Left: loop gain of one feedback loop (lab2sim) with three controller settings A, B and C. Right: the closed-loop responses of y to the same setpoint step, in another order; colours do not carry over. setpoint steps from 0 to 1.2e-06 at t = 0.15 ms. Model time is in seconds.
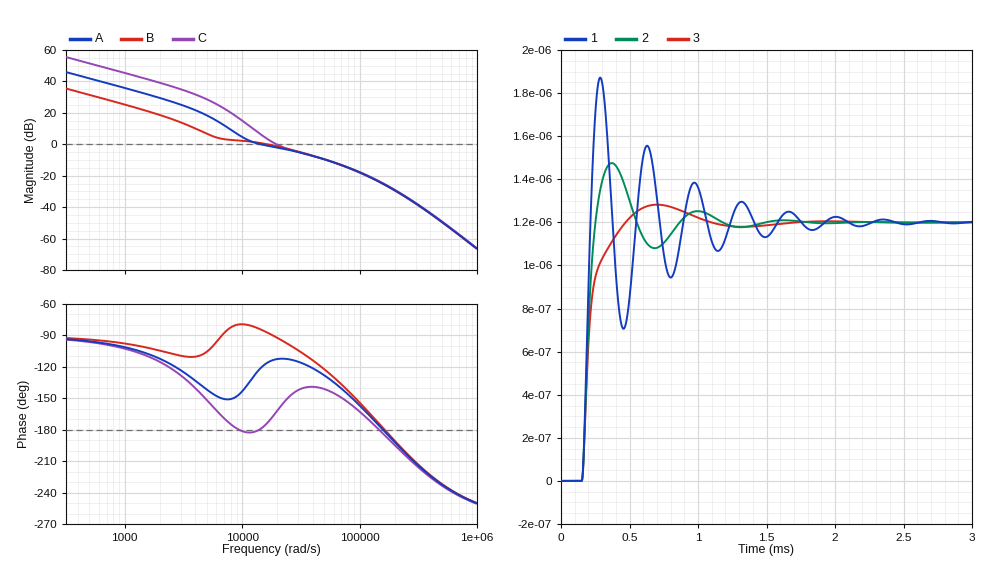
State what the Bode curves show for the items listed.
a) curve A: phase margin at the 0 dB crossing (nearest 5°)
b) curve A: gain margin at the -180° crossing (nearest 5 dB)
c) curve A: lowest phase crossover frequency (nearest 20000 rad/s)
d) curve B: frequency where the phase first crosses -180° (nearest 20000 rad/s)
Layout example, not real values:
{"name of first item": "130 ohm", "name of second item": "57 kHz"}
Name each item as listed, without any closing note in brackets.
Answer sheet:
{"curve A: phase margin at the 0 dB crossing": "60°", "curve A: gain margin at the -180° crossing": "25 dB", "curve A: lowest phase crossover frequency": "160000 rad/s", "curve B: frequency where the phase first crosses -180°": "160000 rad/s"}
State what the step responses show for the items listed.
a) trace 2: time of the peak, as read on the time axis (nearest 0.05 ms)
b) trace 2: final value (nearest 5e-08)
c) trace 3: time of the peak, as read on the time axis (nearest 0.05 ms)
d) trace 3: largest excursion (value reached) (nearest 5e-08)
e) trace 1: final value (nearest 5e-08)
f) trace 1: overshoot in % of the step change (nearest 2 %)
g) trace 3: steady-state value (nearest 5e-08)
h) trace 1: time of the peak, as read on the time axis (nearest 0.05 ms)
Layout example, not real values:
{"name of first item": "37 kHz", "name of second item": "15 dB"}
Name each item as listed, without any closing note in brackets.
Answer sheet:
{"trace 2: time of the peak, as read on the time axis": "0.35 ms", "trace 2: final value": "0.00000120", "trace 3: time of the peak, as read on the time axis": "0.70 ms", "trace 3: largest excursion (value reached)": "0.00000130", "trace 1: final value": "0.00000120", "trace 1: overshoot in % of the step change": "56 %", "trace 3: steady-state value": "0.00000120", "trace 1: time of the peak, as read on the time axis": "0.30 ms"}
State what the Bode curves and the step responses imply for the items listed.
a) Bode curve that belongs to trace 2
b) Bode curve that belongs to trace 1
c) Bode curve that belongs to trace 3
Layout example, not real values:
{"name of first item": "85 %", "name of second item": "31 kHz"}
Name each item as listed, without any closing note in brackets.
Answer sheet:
{"Bode curve that belongs to trace 2": "A", "Bode curve that belongs to trace 1": "C", "Bode curve that belongs to trace 3": "B"}
